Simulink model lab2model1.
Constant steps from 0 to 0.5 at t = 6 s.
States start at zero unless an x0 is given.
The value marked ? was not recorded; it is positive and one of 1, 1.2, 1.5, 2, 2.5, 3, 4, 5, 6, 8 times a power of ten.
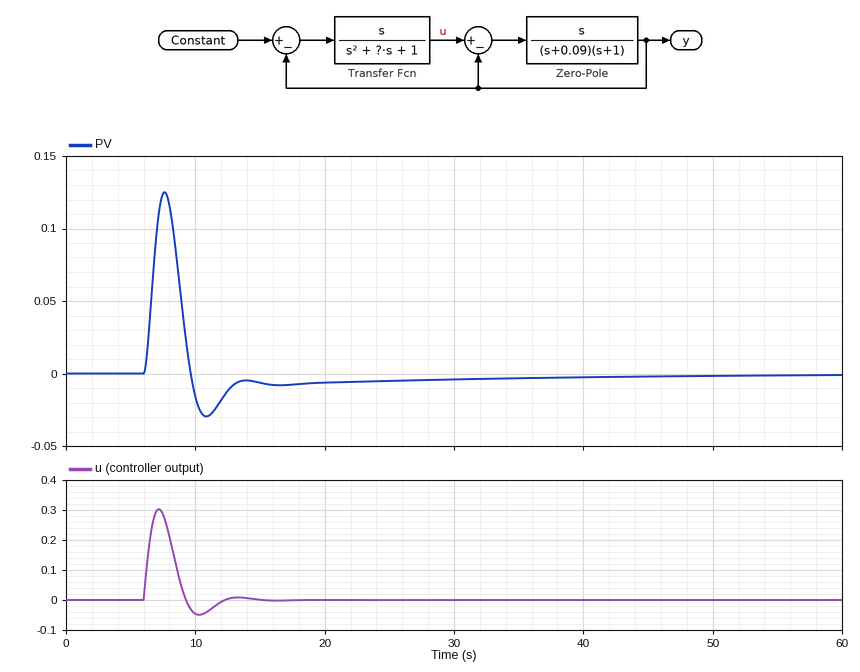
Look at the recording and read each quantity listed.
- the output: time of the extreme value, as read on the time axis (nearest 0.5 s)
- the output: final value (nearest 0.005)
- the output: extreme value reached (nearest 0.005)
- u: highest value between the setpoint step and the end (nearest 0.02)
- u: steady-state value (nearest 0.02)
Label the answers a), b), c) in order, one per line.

a) 7.5 s
b) 0.000
c) 0.125
d) 0.30
e) 0.00
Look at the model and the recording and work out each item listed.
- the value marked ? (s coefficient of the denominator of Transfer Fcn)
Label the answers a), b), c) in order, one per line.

a) 0.5
